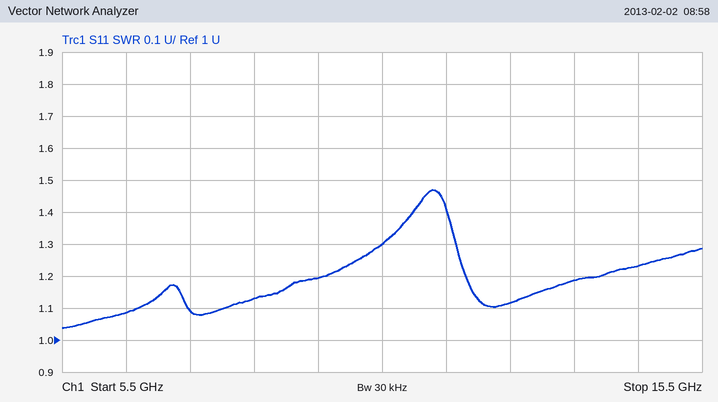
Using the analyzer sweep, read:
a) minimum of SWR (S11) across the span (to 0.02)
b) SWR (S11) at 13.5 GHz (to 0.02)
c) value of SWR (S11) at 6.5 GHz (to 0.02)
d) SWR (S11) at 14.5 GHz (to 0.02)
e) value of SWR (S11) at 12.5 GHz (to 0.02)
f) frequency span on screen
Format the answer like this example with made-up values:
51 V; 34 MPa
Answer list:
1.04; 1.18; 1.08; 1.24; 1.12; 10 GHz
